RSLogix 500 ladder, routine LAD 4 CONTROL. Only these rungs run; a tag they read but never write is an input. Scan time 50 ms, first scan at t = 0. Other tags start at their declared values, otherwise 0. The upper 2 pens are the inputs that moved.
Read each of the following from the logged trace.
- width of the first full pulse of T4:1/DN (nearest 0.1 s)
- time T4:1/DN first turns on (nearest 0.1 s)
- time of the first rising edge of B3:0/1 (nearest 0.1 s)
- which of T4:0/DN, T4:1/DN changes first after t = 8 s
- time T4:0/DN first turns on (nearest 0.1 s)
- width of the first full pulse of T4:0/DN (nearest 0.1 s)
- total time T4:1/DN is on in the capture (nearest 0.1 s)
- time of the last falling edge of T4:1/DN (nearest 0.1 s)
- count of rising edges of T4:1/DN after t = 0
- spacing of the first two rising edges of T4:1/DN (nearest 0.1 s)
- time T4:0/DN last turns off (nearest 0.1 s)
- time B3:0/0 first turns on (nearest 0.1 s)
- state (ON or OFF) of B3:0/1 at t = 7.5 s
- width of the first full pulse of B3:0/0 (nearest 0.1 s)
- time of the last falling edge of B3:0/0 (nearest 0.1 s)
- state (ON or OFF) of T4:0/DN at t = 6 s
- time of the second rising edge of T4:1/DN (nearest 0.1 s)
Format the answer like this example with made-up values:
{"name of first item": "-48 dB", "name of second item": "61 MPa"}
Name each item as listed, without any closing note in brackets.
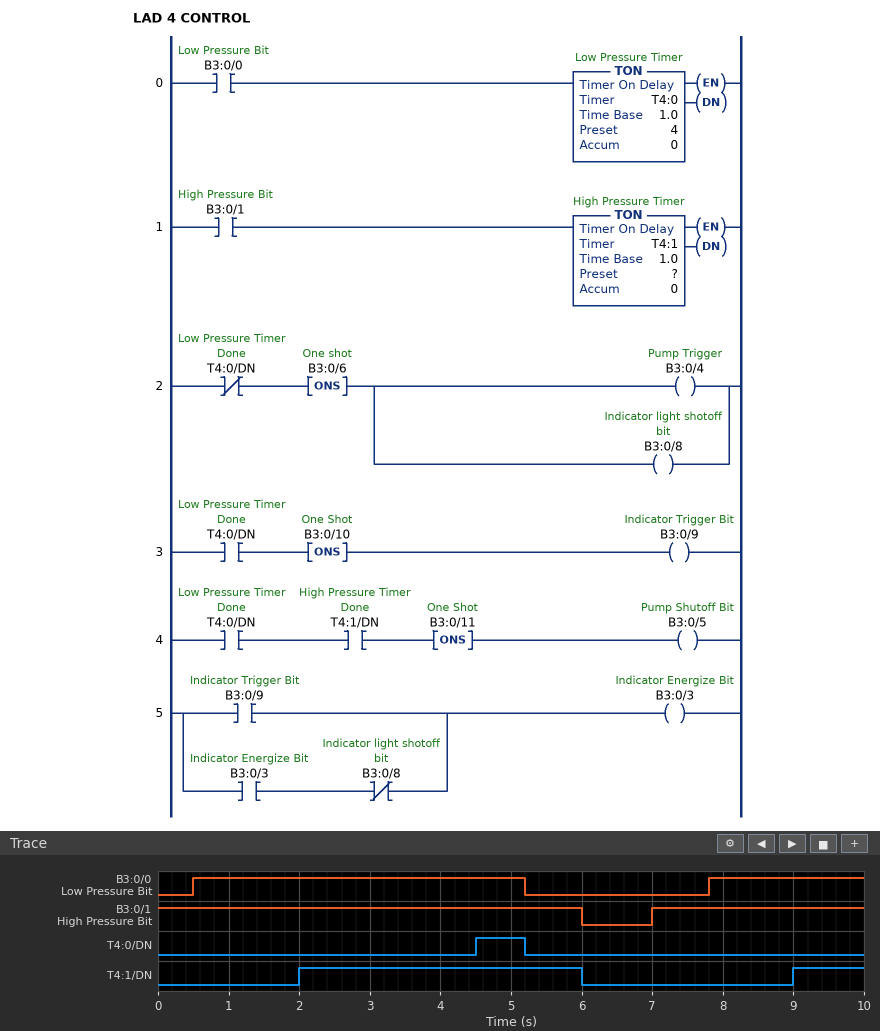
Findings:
{"width of the first full pulse of T4:1/DN": "4.0 s", "time T4:1/DN first turns on": "2.0 s", "time of the first rising edge of B3:0/1": "7.0 s", "which of T4:0/DN, T4:1/DN changes first after t = 8 s": "T4:1/DN", "time T4:0/DN first turns on": "4.5 s", "width of the first full pulse of T4:0/DN": "0.7 s", "total time T4:1/DN is on in the capture": "5.0 s", "time of the last falling edge of T4:1/DN": "6.0 s", "count of rising edges of T4:1/DN after t = 0": "2", "spacing of the first two rising edges of T4:1/DN": "7.0 s", "time T4:0/DN last turns off": "5.2 s", "time B3:0/0 first turns on": "0.5 s", "state (ON or OFF) of B3:0/1 at t = 7.5 s": "ON", "width of the first full pulse of B3:0/0": "4.7 s", "time of the last falling edge of B3:0/0": "5.2 s", "state (ON or OFF) of T4:0/DN at t = 6 s": "OFF", "time of the second rising edge of T4:1/DN": "9.0 s"}
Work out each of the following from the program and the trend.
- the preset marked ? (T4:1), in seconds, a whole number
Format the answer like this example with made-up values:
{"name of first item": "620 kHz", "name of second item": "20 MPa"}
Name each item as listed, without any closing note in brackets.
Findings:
{"the preset marked ? (T4:1), in seconds, a whole number": "2 s"}
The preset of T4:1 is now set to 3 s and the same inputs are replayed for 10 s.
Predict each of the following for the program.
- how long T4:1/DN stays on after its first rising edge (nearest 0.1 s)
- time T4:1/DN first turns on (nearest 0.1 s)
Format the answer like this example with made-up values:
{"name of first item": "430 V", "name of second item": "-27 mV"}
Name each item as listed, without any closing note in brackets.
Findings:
{"how long T4:1/DN stays on after its first rising edge": "3.0 s", "time T4:1/DN first turns on": "3.0 s"}
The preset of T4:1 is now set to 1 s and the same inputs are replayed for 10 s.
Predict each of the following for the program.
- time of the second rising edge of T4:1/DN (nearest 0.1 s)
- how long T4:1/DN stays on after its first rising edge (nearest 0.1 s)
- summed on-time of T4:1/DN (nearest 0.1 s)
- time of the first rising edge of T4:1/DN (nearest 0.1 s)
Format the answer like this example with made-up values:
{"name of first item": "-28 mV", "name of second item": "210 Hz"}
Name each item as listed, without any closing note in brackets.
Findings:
{"time of the second rising edge of T4:1/DN": "8.0 s", "how long T4:1/DN stays on after its first rising edge": "5.0 s", "summed on-time of T4:1/DN": "7.0 s", "time of the first rising edge of T4:1/DN": "1.0 s"}
